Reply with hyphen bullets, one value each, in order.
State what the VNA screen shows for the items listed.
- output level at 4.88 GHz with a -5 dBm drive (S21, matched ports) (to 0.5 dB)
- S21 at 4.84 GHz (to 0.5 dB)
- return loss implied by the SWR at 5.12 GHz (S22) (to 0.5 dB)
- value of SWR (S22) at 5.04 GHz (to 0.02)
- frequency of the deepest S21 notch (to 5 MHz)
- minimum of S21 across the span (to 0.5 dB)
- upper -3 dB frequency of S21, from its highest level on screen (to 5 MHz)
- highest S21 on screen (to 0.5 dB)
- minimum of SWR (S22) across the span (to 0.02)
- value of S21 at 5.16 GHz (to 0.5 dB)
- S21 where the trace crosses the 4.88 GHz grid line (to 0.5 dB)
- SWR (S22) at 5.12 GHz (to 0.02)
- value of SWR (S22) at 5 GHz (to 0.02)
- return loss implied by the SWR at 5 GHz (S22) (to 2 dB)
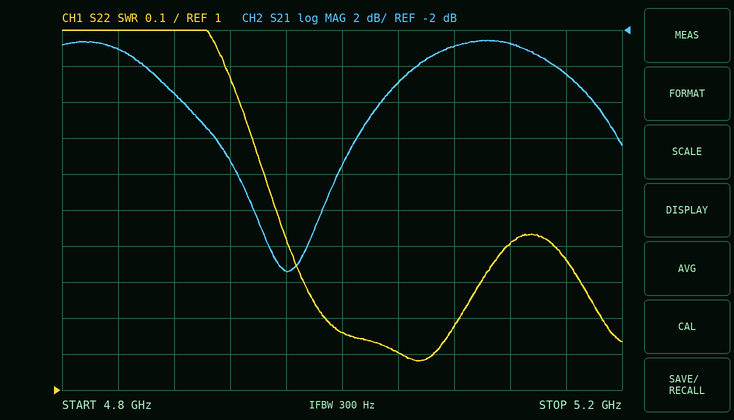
- -10.5 dBm
- -3.0 dB
- 15.5 dB
- 1.10
- 4.960 GHz
- -15.5 dB
- 5.175 GHz
- -2.5 dB
- 1.08
- -4.5 dB
- -5.5 dB
- 1.40
- 1.16
- 22 dB
